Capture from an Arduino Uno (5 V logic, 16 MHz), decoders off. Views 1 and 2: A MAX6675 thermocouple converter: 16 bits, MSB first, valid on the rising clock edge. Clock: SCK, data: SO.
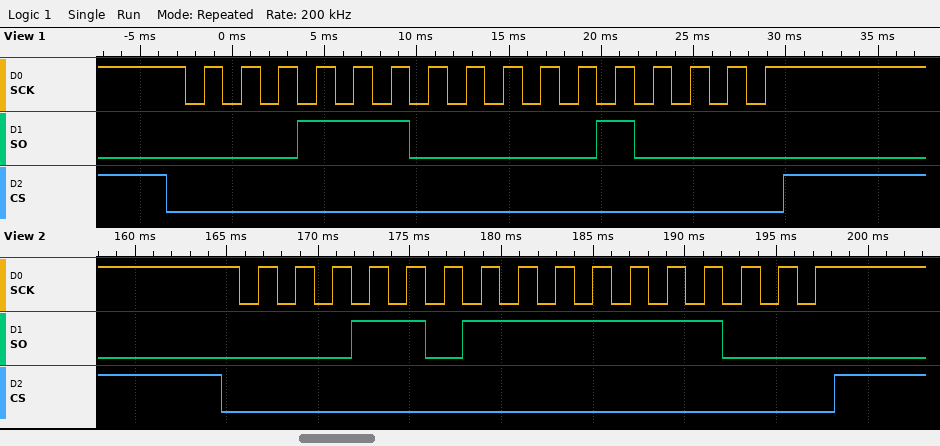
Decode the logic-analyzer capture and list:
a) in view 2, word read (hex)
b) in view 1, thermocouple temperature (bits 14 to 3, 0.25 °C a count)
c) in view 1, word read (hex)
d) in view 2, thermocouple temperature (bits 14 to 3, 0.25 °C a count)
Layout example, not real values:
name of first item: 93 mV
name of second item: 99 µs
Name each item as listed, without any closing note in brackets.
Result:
in view 2, word read: 0x1BF8
in view 1, thermocouple temperature: 224.50 °C
in view 1, word read: 0x1C10
in view 2, thermocouple temperature: 223.75 °C
